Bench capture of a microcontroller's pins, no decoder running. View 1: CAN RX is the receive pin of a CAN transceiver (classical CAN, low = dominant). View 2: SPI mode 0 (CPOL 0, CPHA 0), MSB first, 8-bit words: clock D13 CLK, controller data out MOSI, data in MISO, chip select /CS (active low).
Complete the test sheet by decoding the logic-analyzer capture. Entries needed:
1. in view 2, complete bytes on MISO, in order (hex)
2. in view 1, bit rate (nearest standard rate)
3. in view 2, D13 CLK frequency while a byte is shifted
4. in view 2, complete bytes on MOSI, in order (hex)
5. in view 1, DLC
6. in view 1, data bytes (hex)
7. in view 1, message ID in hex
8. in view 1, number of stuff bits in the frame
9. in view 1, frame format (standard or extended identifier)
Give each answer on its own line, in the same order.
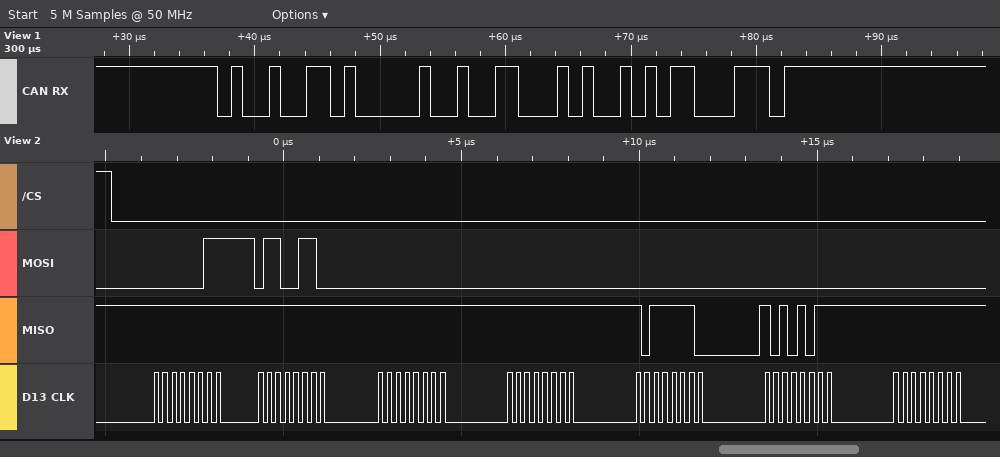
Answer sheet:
FF FF FF FF BE AB FF
1000 kbit/s
4 MHz
03 66 00 00 00 00 00
1
31
0x49A
1
standard
